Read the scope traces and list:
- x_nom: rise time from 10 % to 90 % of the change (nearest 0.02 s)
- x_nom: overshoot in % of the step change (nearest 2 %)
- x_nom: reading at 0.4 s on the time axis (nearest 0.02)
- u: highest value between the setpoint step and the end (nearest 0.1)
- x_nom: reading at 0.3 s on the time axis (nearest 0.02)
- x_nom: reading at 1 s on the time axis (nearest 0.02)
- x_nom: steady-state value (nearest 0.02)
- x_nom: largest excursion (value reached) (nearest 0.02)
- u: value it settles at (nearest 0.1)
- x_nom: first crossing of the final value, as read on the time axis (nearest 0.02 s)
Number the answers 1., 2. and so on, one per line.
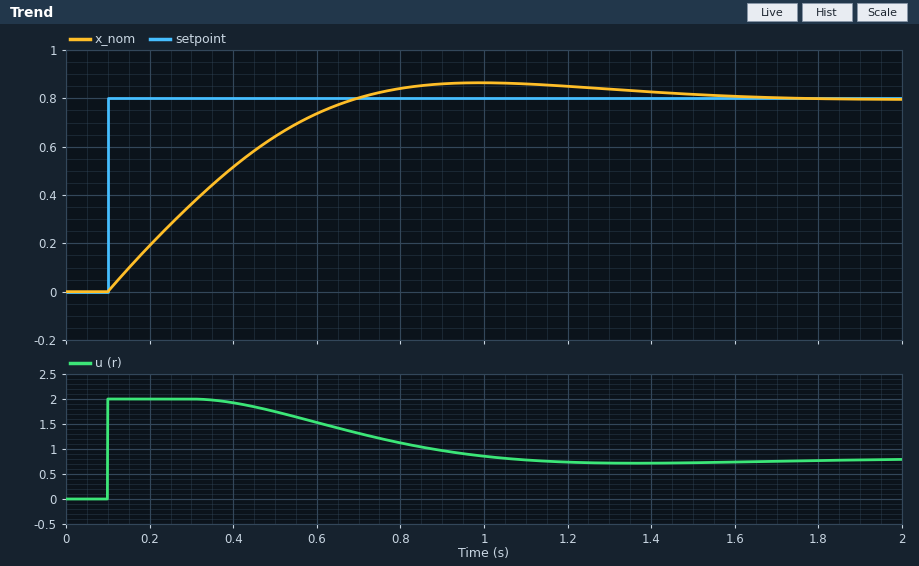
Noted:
1. 0.44 s
2. 8 %
3. 0.52
4. 2.0
5. 0.36
6. 0.86
7. 0.80
8. 0.86
9. 0.8
10. 0.70 s
